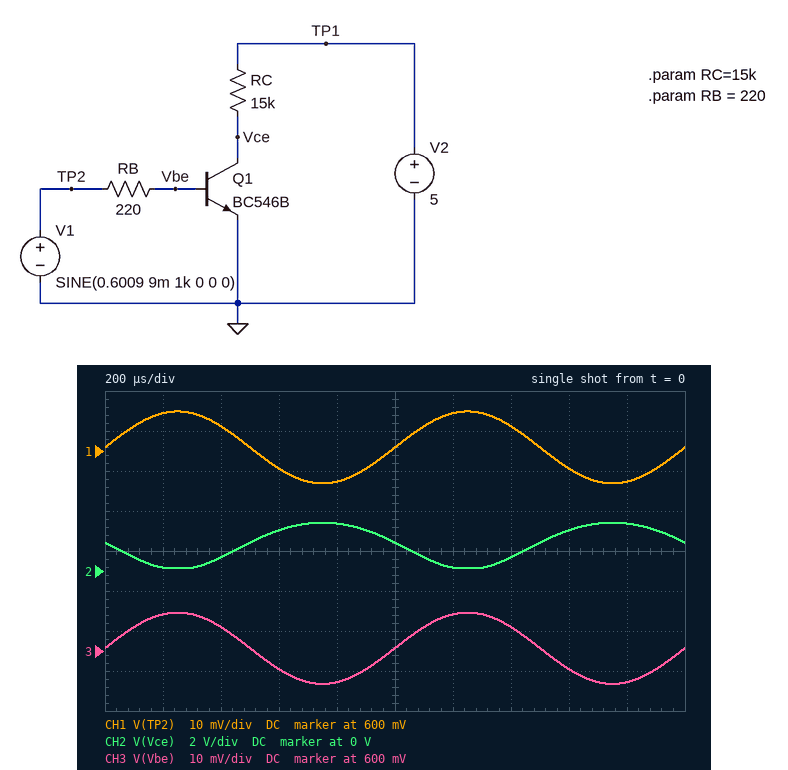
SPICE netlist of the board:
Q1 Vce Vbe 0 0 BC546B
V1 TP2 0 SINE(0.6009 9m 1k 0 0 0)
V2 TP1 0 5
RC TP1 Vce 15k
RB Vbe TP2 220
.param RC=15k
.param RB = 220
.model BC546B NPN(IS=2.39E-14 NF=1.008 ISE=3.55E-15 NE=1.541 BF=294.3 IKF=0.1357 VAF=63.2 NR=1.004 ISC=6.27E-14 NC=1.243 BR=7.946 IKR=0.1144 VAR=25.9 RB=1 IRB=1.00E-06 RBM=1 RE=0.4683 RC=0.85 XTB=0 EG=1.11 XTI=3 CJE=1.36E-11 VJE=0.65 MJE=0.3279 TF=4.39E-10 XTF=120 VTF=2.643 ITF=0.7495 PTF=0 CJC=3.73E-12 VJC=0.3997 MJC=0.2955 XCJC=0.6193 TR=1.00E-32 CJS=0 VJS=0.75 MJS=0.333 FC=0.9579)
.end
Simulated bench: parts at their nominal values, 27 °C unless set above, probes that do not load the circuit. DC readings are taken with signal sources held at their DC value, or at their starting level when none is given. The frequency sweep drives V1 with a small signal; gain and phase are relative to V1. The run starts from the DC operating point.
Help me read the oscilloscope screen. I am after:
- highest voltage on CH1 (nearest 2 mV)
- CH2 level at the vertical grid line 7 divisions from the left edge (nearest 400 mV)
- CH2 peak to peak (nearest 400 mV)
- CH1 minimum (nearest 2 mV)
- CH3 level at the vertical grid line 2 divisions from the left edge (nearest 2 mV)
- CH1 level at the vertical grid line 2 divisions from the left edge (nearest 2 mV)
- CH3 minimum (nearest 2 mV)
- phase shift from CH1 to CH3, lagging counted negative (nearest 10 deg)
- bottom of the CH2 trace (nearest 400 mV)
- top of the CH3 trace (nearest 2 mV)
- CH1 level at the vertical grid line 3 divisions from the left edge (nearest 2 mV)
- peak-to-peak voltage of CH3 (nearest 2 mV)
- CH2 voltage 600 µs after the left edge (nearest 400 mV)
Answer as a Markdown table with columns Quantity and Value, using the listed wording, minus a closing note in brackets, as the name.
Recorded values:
| Quantity | Value |
|---|---|
| highest voltage on CH1 | 610 mV |
| CH2 level at the vertical grid line 7 divisions from the left edge | 800 mV |
| CH2 peak to peak | 2.4 V |
| CH1 minimum | 592 mV |
| CH3 level at the vertical grid line 2 divisions from the left edge | 606 mV |
| CH1 level at the vertical grid line 2 divisions from the left edge | 606 mV |
| CH3 minimum | 592 mV |
| phase shift from CH1 to CH3, lagging counted negative | 0 deg |
| bottom of the CH2 trace | 0 V |
| top of the CH3 trace | 610 mV |
| CH1 level at the vertical grid line 3 divisions from the left edge | 596 mV |
| peak-to-peak voltage of CH3 | 18 mV |
| CH2 voltage 600 µs after the left edge | 2.0 V |
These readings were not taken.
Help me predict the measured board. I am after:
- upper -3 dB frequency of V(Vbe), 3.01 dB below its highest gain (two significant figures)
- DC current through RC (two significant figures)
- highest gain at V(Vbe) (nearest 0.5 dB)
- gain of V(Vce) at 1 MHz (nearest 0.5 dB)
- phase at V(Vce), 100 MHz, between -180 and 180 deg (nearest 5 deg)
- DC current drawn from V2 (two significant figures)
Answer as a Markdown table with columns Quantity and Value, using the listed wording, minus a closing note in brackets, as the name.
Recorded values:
| Quantity | Value |
|---|---|
| upper -3 dB frequency of V(Vbe), 3.01 dB below its highest gain | 1.5 MHz |
| DC current through RC | 240 µA |
| highest gain at V(Vbe) | 0 dB |
| gain of V(Vce) at 1 MHz | 40.0 dB |
| phase at V(Vce), 100 MHz, between -180 and 180 deg | 25 deg |
| DC current drawn from V2 | 240 µA |
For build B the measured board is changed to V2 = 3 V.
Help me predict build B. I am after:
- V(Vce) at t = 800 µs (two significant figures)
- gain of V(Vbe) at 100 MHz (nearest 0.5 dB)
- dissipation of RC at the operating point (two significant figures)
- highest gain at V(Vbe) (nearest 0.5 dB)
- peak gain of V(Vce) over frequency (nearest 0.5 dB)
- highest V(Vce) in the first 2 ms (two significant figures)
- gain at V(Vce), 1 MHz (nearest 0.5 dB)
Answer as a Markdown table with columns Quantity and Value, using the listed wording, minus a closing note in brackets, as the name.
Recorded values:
| Quantity | Value |
|---|---|
| V(Vce) at t = 800 µs | 450 mV |
| gain of V(Vbe) at 100 MHz | -15.0 dB |
| dissipation of RC at the operating point | 580 µW |
| highest gain at V(Vbe) | -2.0 dB |
| peak gain of V(Vce) over frequency | 14.0 dB |
| highest V(Vce) in the first 2 ms | 490 mV |
| gain at V(Vce), 1 MHz | 13.0 dB |
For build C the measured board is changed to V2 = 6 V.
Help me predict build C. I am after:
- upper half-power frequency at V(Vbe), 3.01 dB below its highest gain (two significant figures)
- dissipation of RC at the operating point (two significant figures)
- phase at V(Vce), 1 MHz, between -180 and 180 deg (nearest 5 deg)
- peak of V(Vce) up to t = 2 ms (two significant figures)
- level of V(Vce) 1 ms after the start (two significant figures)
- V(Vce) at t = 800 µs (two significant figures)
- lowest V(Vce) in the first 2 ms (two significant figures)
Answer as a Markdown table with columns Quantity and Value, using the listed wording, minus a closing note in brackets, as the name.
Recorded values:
| Quantity | Value |
|---|---|
| upper half-power frequency at V(Vbe), 3.01 dB below its highest gain | 1.7 MHz |
| dissipation of RC at the operating point | 880 µW |
| phase at V(Vce), 1 MHz, between -180 and 180 deg | 145 deg |
| peak of V(Vce) up to t = 2 ms | 3.4 V |
| level of V(Vce) 1 ms after the start | 2.4 V |
| V(Vce) at t = 800 µs | 3.3 V |
| lowest V(Vce) in the first 2 ms | 1.0 V |
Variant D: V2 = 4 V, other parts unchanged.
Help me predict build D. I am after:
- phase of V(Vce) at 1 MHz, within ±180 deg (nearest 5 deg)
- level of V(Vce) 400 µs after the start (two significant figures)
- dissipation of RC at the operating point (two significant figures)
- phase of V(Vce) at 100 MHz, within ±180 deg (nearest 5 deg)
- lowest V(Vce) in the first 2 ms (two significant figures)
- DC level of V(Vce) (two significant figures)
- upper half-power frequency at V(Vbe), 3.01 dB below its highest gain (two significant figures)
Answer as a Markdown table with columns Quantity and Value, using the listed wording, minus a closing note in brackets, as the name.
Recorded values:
| Quantity | Value |
|---|---|
| phase of V(Vce) at 1 MHz, within ±180 deg | 130 deg |
| level of V(Vce) 400 µs after the start | 79 mV |
| dissipation of RC at the operating point | 830 µW |
| phase of V(Vce) at 100 MHz, within ±180 deg | 15 deg |
| lowest V(Vce) in the first 2 ms | 56 mV |
| DC level of V(Vce) | 470 mV |
| upper half-power frequency at V(Vbe), 3.01 dB below its highest gain | 990 kHz |
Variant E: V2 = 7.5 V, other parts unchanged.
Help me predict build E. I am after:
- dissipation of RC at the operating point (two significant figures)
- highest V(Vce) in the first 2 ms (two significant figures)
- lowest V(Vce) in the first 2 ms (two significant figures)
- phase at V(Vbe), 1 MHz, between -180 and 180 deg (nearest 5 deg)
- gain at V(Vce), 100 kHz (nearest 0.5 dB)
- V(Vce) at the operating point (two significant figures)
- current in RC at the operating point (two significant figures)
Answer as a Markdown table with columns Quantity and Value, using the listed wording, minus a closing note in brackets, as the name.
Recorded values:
| Quantity | Value |
|---|---|
| dissipation of RC at the operating point | 920 µW |
| highest V(Vce) in the first 2 ms | 4.8 V |
| lowest V(Vce) in the first 2 ms | 2.4 V |
| phase at V(Vbe), 1 MHz, between -180 and 180 deg | -20 deg |
| gain at V(Vce), 100 kHz | 42.5 dB |
| V(Vce) at the operating point | 3.8 V |
| current in RC at the operating point | 250 µA |
